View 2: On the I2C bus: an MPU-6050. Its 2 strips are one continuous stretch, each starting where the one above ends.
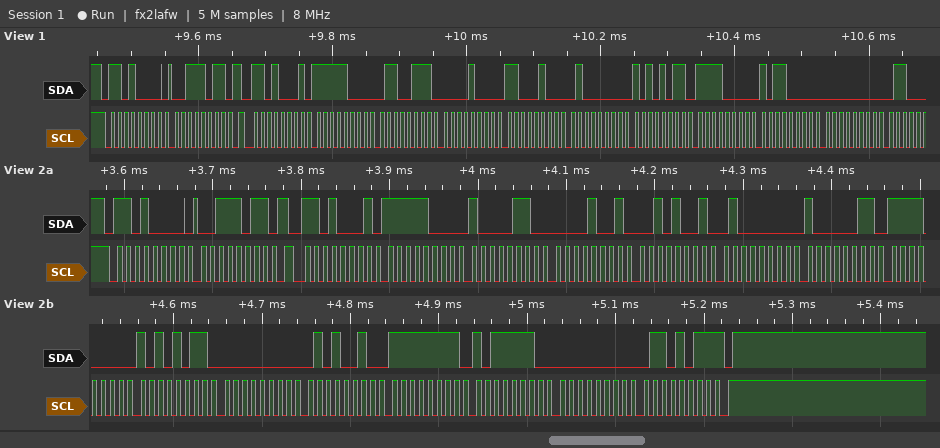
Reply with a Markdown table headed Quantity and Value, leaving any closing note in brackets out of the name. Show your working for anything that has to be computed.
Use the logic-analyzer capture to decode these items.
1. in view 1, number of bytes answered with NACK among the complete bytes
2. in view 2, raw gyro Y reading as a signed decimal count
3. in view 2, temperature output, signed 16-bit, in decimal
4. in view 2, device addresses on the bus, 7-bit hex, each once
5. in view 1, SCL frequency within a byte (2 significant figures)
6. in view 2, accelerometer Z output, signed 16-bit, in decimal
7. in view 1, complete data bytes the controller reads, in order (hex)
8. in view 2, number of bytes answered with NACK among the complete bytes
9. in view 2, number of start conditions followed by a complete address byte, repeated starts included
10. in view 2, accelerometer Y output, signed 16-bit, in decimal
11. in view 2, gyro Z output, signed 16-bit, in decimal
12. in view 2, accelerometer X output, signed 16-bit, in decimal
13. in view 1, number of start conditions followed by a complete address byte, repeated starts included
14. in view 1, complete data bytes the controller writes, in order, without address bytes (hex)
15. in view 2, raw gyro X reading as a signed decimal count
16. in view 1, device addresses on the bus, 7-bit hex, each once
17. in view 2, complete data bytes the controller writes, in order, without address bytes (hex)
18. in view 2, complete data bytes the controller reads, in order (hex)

| Quantity | Value |
|---|---|
| in view 1, number of bytes answered with NACK among the complete bytes | 0 |
| in view 2, raw gyro Y reading as a signed decimal count | 0xFFBE = -66 |
| in view 2, temperature output, signed 16-bit, in decimal | 0xF0AB = -3925 |
| in view 2, device addresses on the bus, 7-bit hex, each once | 0x68 |
| in view 1, SCL frequency within a byte | 100 kHz |
| in view 2, accelerometer Z output, signed 16-bit, in decimal | 0x4083 = 16515 |
| in view 1, complete data bytes the controller reads, in order | F8 67 08 C4 40 AB F0 B0 00 |
| in view 2, number of bytes answered with NACK among the complete bytes | 1 |
| in view 2, number of start conditions followed by a complete address byte, repeated starts included | 2 |
| in view 2, accelerometer Y output, signed 16-bit, in decimal | 0x0929 = 2345 |
| in view 2, gyro Z output, signed 16-bit, in decimal | 0x006B = 107 |
| in view 2, accelerometer X output, signed 16-bit, in decimal | 0xF886 = -1914 |
| in view 1, number of start conditions followed by a complete address byte, repeated starts included | 2 |
| in view 1, complete data bytes the controller writes, in order, without address bytes | 3B |
| in view 2, raw gyro X reading as a signed decimal count | 0x0052 = 82 |
| in view 1, device addresses on the bus, 7-bit hex, each once | 0x68 |
| in view 2, complete data bytes the controller writes, in order, without address bytes | 3B |
| in view 2, complete data bytes the controller reads, in order | F8 86 09 29 40 83 F0 AB 00 52 FF BE 00 6B |
